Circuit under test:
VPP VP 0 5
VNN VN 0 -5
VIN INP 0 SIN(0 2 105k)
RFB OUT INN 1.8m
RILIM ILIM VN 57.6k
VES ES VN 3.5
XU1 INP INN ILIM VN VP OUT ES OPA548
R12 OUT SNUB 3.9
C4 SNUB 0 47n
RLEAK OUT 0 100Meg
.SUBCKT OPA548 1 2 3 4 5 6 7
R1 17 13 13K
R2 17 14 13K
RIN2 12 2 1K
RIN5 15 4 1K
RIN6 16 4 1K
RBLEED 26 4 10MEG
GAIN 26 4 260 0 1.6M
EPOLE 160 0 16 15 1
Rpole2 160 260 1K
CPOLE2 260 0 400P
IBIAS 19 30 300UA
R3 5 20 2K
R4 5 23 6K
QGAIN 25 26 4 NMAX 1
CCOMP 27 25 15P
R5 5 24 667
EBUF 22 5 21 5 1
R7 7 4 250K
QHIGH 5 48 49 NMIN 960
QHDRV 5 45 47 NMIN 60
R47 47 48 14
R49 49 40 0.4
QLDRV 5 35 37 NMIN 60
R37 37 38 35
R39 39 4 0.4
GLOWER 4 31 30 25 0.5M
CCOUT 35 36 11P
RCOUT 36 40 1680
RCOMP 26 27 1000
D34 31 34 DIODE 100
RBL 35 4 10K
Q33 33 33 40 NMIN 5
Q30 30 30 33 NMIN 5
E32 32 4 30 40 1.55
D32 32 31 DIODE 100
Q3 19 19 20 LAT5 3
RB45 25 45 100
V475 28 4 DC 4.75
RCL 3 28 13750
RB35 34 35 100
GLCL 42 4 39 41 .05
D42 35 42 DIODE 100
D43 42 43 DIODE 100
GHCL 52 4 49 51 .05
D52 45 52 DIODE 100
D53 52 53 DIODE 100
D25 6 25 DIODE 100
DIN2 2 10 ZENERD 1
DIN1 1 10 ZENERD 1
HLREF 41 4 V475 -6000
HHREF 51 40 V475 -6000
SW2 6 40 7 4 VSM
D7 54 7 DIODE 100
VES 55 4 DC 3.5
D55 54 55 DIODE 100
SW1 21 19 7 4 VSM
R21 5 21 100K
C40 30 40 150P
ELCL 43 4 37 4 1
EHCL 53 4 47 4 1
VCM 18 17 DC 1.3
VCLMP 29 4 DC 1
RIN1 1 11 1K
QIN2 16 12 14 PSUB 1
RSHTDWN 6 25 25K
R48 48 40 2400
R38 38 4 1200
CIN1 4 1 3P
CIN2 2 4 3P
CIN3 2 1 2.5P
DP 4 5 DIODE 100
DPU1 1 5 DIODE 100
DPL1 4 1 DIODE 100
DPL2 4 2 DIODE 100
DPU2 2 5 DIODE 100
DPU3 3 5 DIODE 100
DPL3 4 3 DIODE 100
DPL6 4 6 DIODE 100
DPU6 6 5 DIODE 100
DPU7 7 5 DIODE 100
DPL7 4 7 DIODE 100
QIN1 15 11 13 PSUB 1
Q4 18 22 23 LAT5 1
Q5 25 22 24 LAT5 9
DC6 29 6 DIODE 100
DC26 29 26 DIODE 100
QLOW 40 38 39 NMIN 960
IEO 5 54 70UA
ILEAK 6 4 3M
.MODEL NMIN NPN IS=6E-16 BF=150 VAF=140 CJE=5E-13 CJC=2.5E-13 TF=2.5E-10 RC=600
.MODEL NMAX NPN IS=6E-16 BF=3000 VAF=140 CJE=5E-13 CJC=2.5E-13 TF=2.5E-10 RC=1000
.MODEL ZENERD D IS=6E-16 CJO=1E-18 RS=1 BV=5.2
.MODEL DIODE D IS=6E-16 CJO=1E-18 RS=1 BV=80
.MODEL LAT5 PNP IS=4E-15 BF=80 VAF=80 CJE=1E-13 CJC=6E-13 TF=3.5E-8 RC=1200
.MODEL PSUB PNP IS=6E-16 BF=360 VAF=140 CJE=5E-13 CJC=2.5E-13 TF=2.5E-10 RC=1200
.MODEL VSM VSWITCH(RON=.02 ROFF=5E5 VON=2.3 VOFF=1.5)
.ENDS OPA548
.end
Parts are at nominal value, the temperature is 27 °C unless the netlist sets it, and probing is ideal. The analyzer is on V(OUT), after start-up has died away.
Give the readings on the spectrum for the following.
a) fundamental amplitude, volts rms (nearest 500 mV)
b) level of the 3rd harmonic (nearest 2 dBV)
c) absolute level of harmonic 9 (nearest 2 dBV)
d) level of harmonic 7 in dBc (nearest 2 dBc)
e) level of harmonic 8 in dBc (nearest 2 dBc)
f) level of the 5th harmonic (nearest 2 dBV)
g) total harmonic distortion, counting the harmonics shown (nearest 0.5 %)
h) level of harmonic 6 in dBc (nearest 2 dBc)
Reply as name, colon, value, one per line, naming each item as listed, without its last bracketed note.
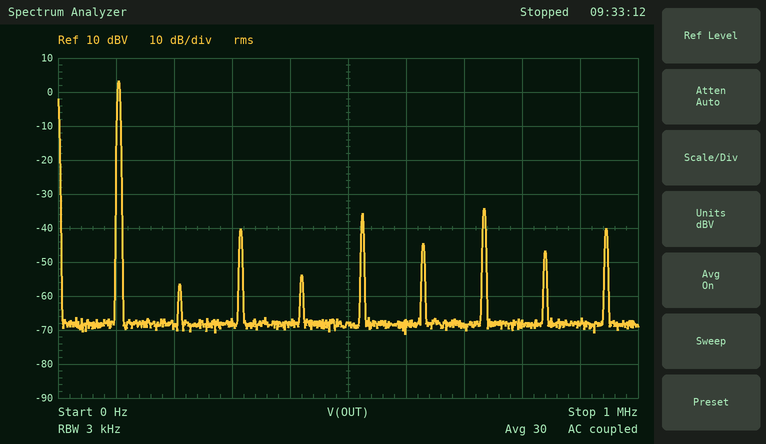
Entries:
fundamental amplitude, volts rms: 1.5 V
level of the 3rd harmonic: -40 dBV
absolute level of harmonic 9: -40 dBV
level of harmonic 7 in dBc: -38 dBc
level of harmonic 8 in dBc: -50 dBc
level of the 5th harmonic: -36 dBV
total harmonic distortion, counting the harmonics shown: 2.0 %
level of harmonic 6 in dBc: -48 dBc
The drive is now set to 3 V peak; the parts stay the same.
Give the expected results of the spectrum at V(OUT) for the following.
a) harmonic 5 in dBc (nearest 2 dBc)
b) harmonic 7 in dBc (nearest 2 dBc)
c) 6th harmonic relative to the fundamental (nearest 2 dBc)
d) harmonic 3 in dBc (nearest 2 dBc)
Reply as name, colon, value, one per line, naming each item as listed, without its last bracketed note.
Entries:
harmonic 5 in dBc: -28 dBc
harmonic 7 in dBc: -32 dBc
6th harmonic relative to the fundamental: -28 dBc
harmonic 3 in dBc: -28 dBc
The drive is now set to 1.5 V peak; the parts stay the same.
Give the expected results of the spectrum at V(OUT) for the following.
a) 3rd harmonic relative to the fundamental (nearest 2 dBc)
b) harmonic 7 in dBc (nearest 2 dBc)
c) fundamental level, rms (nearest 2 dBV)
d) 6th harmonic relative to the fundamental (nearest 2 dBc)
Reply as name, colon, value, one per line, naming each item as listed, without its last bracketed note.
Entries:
3rd harmonic relative to the fundamental: -42 dBc
harmonic 7 in dBc: -36 dBc
fundamental level, rms: 0 dBV
6th harmonic relative to the fundamental: -46 dBc
